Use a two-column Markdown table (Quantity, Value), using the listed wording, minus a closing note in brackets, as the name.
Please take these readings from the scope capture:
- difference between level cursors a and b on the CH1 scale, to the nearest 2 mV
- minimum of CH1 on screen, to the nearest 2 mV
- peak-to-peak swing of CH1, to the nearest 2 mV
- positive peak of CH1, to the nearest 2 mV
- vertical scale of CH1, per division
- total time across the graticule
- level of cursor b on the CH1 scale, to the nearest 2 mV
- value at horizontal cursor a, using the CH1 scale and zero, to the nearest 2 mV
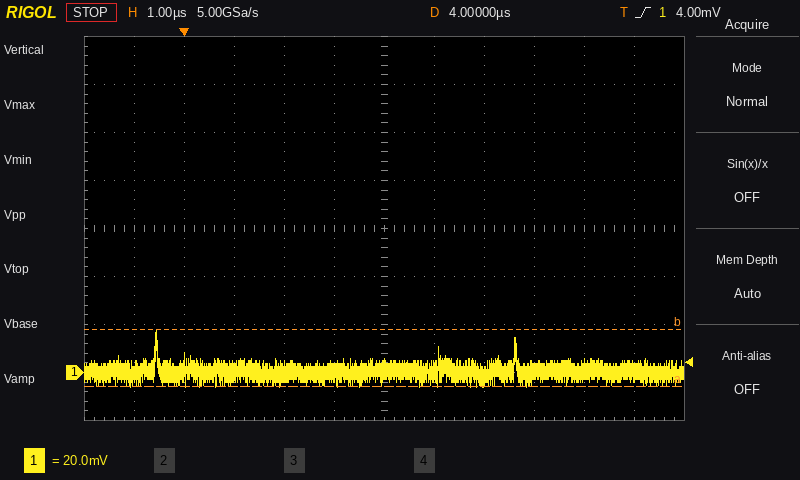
| Quantity | Value |
|---|---|
| difference between level cursors a and b on the CH1 scale, to the nearest 2 mV | 24 mV |
| minimum of CH1 on screen, to the nearest 2 mV | -6 mV |
| peak-to-peak swing of CH1, to the nearest 2 mV | 24 mV |
| positive peak of CH1, to the nearest 2 mV | 18 mV |
| vertical scale of CH1, per division | 20 mV |
| total time across the graticule | 12 µs |
| level of cursor b on the CH1 scale, to the nearest 2 mV | 18 mV |
| value at horizontal cursor a, using the CH1 scale and zero, to the nearest 2 mV | -6 mV |
